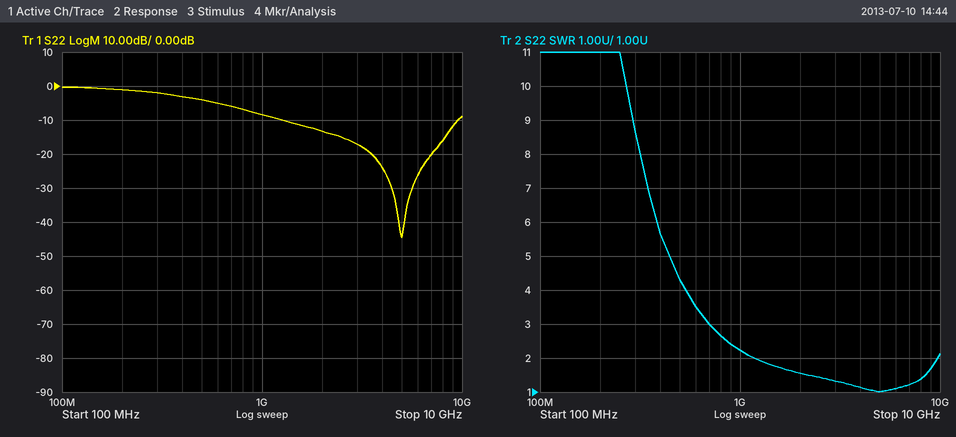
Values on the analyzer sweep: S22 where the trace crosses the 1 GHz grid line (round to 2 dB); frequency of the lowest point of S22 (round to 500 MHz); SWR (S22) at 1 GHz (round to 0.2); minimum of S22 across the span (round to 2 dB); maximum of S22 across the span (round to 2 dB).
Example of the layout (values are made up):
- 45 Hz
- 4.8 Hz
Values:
- -8 dB
- 5.0 GHz
- 2.2
- -44 dB
- 0 dB
